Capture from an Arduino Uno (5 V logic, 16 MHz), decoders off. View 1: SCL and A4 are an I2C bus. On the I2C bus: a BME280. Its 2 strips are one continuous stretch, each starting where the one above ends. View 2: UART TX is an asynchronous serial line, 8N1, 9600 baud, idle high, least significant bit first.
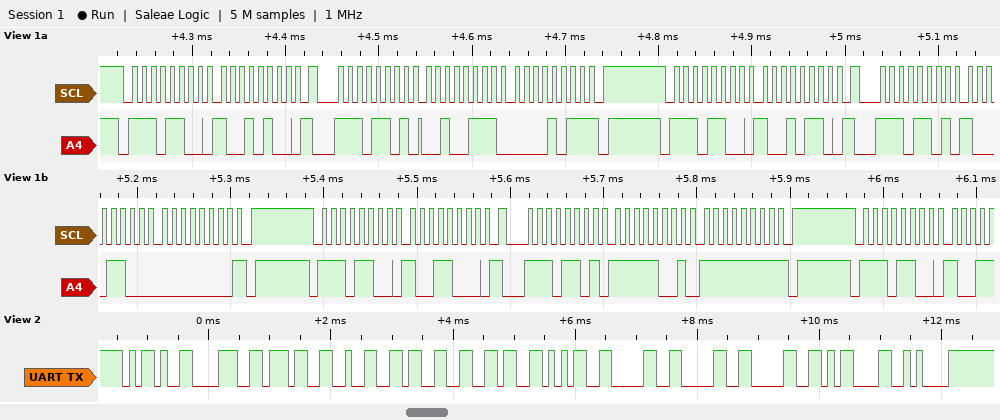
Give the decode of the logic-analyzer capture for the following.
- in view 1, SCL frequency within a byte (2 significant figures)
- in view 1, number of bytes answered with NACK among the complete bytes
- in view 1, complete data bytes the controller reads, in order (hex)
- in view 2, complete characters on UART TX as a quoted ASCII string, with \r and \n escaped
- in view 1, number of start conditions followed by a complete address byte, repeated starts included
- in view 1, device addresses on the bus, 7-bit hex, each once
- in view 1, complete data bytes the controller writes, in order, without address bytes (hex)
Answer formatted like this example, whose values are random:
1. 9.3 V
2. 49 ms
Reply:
1. 100 kHz
2. 3
3. 27 0B 8C 00 F9 FF
4. "-872365000\r\n"
5. 7
6. 0x76
7. 94 96 98
